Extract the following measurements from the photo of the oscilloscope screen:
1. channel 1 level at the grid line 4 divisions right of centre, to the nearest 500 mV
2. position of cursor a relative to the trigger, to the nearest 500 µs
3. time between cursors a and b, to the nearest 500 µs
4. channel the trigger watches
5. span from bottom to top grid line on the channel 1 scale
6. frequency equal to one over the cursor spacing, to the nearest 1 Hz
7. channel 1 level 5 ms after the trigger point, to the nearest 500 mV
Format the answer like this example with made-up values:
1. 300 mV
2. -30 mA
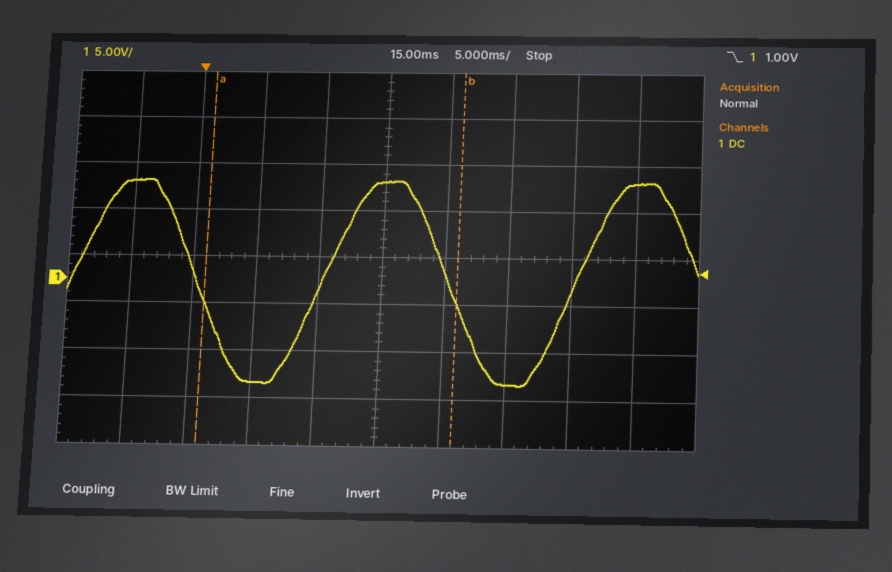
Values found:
1. 10.5 V
2. +1.0 ms
3. 20.0 ms
4. channel 1
5. 40 V
6. 50 Hz
7. -11.0 V
